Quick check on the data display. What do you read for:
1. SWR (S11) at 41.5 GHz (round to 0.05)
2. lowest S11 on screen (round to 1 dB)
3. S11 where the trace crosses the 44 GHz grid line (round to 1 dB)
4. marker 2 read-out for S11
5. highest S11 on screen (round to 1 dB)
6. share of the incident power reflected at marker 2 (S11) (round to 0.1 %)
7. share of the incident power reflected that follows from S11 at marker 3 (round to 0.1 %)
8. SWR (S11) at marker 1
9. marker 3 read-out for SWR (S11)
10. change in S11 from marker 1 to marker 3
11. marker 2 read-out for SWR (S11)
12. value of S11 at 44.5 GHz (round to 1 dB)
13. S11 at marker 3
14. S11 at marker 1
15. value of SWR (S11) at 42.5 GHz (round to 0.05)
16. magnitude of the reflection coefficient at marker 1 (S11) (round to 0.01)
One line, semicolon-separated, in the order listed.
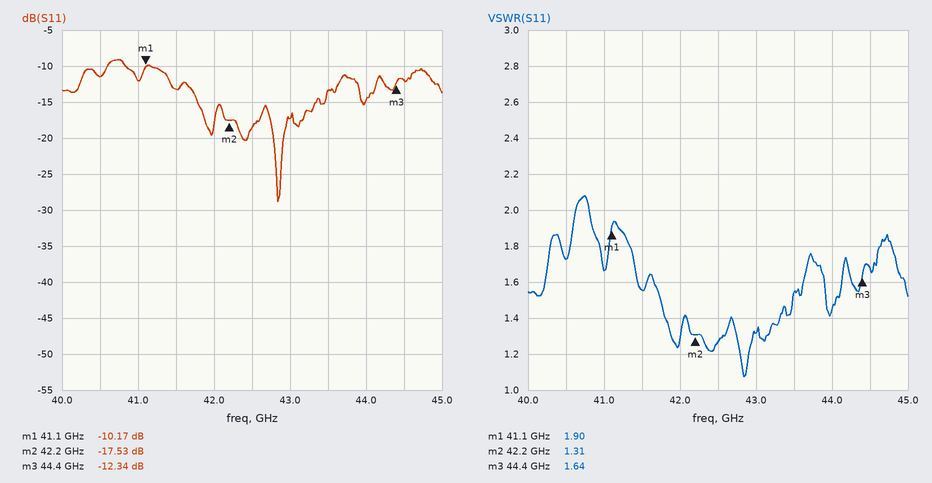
1.55; -29 dB; -15 dB; -17.53 dB; -9 dB; 1.8 %; 5.8 %; 1.90; 1.64; -2.17 dB; 1.31; -12 dB; -12.34 dB; -10.17 dB; 1.25; 0.31
